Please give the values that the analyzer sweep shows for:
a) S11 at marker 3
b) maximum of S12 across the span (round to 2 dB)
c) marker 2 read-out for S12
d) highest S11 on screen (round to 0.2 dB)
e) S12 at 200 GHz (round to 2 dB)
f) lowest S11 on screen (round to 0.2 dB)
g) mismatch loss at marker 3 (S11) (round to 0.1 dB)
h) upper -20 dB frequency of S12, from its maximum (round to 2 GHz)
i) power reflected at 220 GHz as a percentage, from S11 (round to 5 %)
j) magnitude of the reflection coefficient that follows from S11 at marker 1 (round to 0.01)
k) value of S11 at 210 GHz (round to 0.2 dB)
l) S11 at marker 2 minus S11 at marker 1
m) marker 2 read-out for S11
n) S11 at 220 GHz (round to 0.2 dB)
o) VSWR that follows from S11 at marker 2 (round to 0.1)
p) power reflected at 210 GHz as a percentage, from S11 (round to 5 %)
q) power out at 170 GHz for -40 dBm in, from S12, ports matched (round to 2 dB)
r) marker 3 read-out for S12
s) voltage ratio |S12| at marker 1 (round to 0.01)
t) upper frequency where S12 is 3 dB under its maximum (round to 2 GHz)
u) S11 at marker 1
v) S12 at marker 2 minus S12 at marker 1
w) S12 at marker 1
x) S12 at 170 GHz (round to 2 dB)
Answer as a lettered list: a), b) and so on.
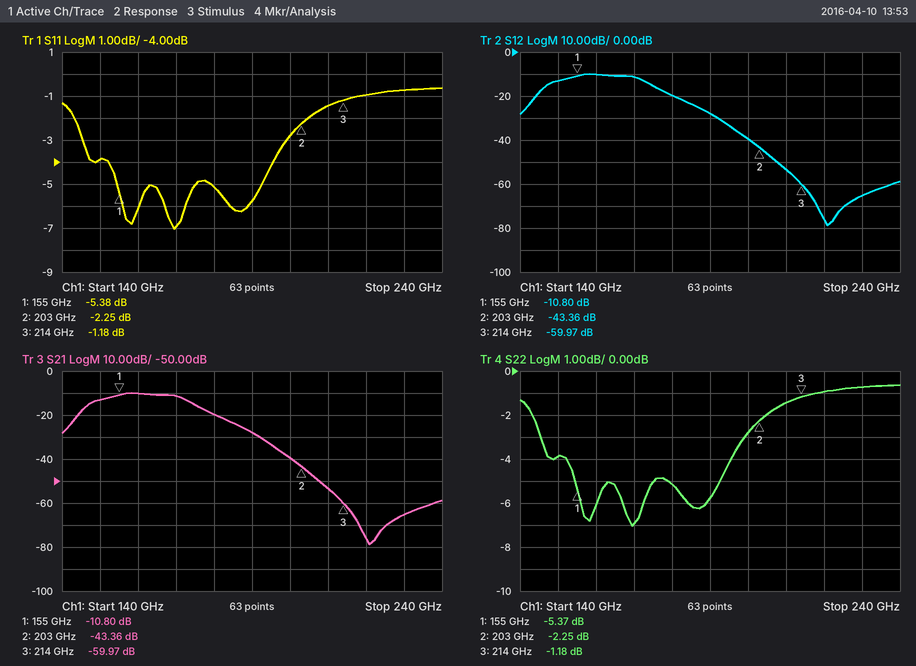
a) -1.18 dB
b) -10 dB
c) -43.36 dB
d) -0.6 dB
e) -40 dB
f) -7.0 dB
g) 6.2 dB
h) 192 GHz
i) 80 %
j) 0.54
k) -1.4 dB
l) 3.13 dB
m) -2.25 dB
n) -1.0 dB
o) 7.8
p) 70 %
q) -52 dBm
r) -59.97 dB
s) 0.29
t) 172 GHz
u) -5.38 dB
v) -32.56 dB
w) -10.80 dB
x) -12 dB
